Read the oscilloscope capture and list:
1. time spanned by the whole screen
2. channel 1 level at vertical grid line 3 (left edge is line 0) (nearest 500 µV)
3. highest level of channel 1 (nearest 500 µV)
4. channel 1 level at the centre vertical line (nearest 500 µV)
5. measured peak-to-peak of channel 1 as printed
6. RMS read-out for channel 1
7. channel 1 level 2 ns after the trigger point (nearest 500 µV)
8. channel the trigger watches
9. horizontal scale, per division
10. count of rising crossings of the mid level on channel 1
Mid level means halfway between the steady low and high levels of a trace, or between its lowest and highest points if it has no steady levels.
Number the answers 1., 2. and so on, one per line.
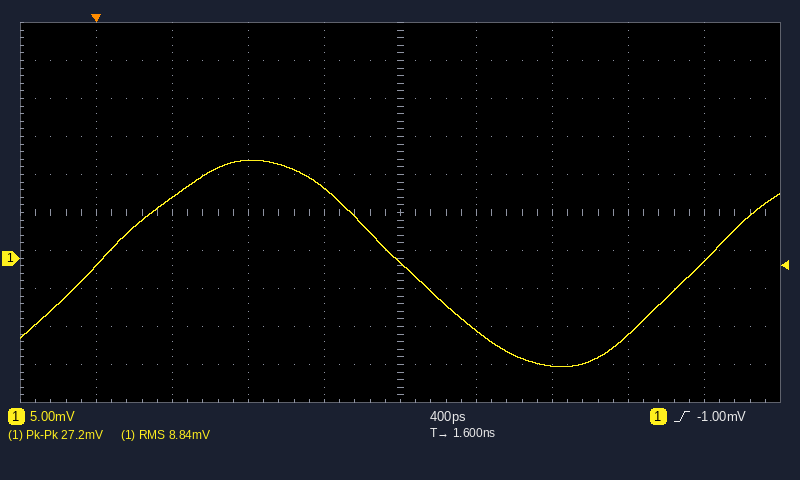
1. 4 ns
2. 13.0 mV
3. 13.0 mV
4. -500 µV
5. 27.2 mV
6. 8.84 mV
7. -9.5 mV
8. channel 1
9. 400 ps
10. 2
